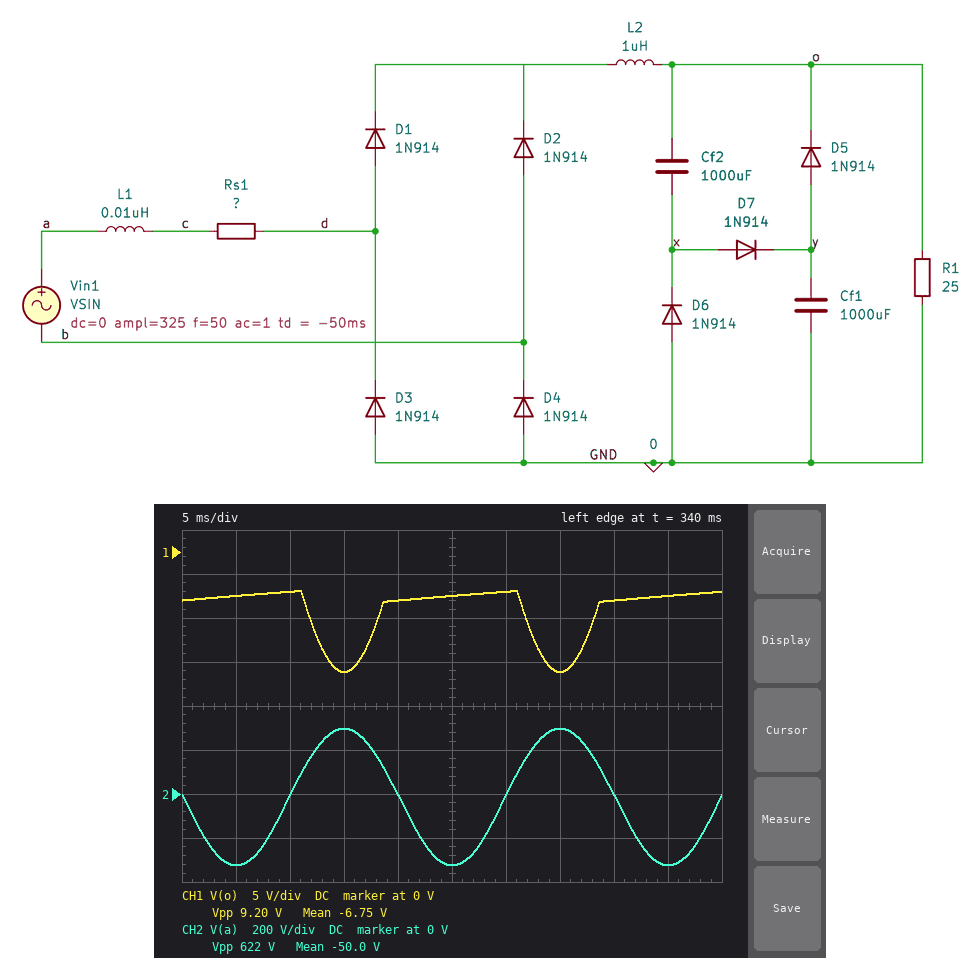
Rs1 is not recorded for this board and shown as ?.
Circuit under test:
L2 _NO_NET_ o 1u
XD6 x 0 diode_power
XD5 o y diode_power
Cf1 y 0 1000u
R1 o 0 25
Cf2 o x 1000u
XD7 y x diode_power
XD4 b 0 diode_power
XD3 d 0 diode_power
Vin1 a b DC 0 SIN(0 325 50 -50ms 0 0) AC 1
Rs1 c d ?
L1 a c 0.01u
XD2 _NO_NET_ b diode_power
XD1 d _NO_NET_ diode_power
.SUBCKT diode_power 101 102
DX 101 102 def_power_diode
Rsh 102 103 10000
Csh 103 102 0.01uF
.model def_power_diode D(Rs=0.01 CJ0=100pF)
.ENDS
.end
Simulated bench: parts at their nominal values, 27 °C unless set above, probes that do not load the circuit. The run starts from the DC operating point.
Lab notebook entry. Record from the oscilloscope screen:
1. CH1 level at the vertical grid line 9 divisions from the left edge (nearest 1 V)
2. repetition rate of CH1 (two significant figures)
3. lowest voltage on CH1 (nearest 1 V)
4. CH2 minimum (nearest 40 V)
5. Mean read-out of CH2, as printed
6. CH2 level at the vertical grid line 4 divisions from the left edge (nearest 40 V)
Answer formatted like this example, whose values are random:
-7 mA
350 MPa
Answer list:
-5 V
50 Hz
-14 V
-320 V
-50.0 V
0 V
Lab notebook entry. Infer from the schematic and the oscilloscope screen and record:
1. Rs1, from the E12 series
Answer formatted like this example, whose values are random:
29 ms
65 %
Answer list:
0.22 Ω
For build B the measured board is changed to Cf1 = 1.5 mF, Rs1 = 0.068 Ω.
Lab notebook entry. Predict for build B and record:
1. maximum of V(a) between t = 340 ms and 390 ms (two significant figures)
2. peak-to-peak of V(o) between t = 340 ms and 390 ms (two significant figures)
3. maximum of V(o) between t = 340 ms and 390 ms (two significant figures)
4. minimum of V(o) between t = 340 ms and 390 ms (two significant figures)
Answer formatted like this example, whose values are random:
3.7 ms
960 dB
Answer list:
250 V
23 V
-14 V
-37 V
